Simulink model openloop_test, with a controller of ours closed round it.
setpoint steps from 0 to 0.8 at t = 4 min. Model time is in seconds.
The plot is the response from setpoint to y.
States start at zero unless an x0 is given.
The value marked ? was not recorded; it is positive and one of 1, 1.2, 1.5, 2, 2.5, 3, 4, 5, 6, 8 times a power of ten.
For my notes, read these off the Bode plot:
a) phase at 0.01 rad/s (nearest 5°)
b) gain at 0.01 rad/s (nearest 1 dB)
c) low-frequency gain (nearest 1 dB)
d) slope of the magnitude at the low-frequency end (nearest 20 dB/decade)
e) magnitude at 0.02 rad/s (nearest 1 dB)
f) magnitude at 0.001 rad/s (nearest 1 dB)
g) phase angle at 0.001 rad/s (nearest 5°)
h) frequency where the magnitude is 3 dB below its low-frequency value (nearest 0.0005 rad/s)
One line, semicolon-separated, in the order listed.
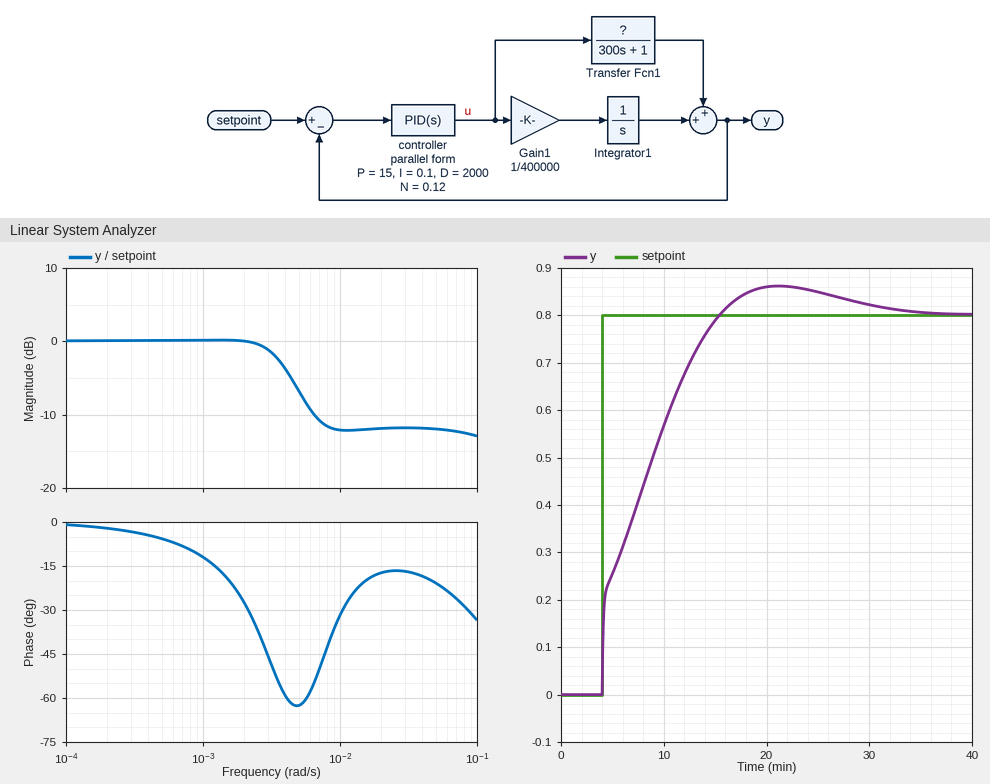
-30°; -12 dB; 0 dB; 0 dB/decade; -12 dB; 0 dB; -10°; 0.0035 rad/s
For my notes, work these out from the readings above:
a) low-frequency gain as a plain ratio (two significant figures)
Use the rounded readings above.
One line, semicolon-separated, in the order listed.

1.0
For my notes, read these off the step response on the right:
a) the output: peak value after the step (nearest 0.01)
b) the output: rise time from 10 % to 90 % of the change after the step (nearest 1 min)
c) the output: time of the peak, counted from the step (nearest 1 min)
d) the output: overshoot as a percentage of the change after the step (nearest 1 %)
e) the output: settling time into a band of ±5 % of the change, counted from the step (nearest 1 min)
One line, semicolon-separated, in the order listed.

0.86; 9 min; 17 min; 7 %; 22 min
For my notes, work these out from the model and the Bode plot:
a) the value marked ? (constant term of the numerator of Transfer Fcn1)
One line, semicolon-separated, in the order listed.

0.05
